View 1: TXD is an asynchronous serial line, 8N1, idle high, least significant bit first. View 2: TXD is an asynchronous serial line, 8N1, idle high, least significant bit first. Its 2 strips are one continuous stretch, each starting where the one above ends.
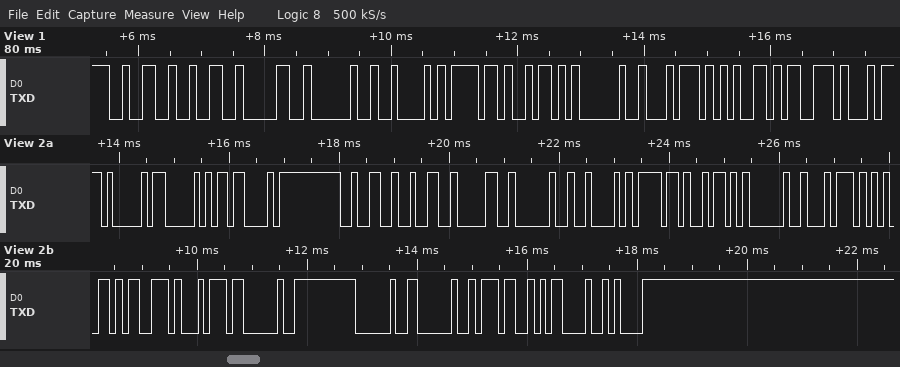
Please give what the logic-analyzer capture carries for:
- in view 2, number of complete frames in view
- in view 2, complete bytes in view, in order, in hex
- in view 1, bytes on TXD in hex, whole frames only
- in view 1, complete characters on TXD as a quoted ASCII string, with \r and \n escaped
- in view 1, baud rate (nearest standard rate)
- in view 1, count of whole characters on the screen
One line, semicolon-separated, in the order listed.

21; 0x41 0x50 0x43 0x32 0x32 0x30 0x20 0x42 0x6F 0x5A 0x20 0x74 0x65 0x73 0x74 0x20 0x20 0x20 0x37 0x0D 0x0A; 32 32 30 20 42 6F 5A 20 74 65 73; "220 BoZ tes"; 9600 baud; 11
